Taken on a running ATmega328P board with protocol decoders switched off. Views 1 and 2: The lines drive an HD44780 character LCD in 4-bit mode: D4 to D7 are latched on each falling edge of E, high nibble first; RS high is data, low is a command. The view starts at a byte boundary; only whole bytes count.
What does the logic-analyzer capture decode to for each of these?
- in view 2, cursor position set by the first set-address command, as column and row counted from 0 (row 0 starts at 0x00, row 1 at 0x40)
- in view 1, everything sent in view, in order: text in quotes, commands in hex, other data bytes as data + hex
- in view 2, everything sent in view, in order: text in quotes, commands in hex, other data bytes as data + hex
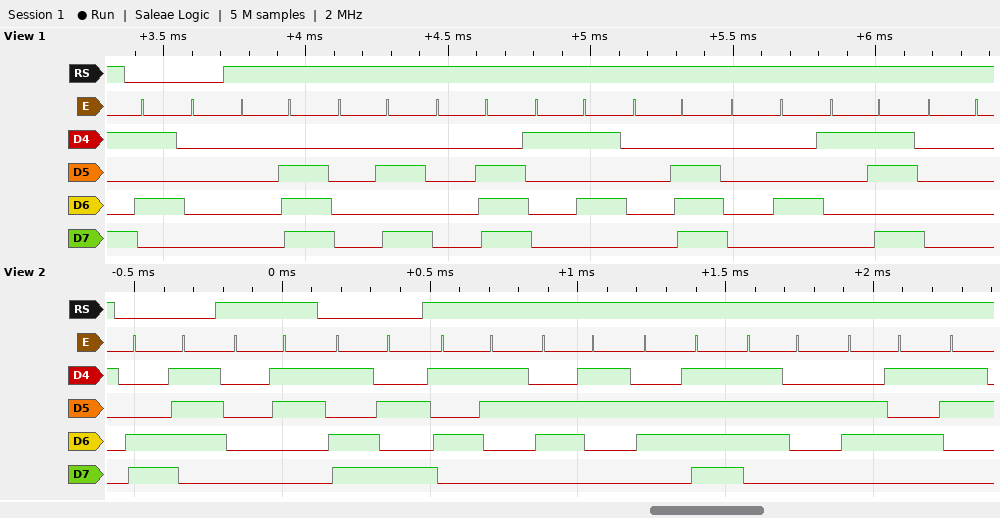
column 7, row 1
0x50 data 0E 0A 0E 15 0E 04 1B 00
0xC7 data 03 0xDA "Score"
